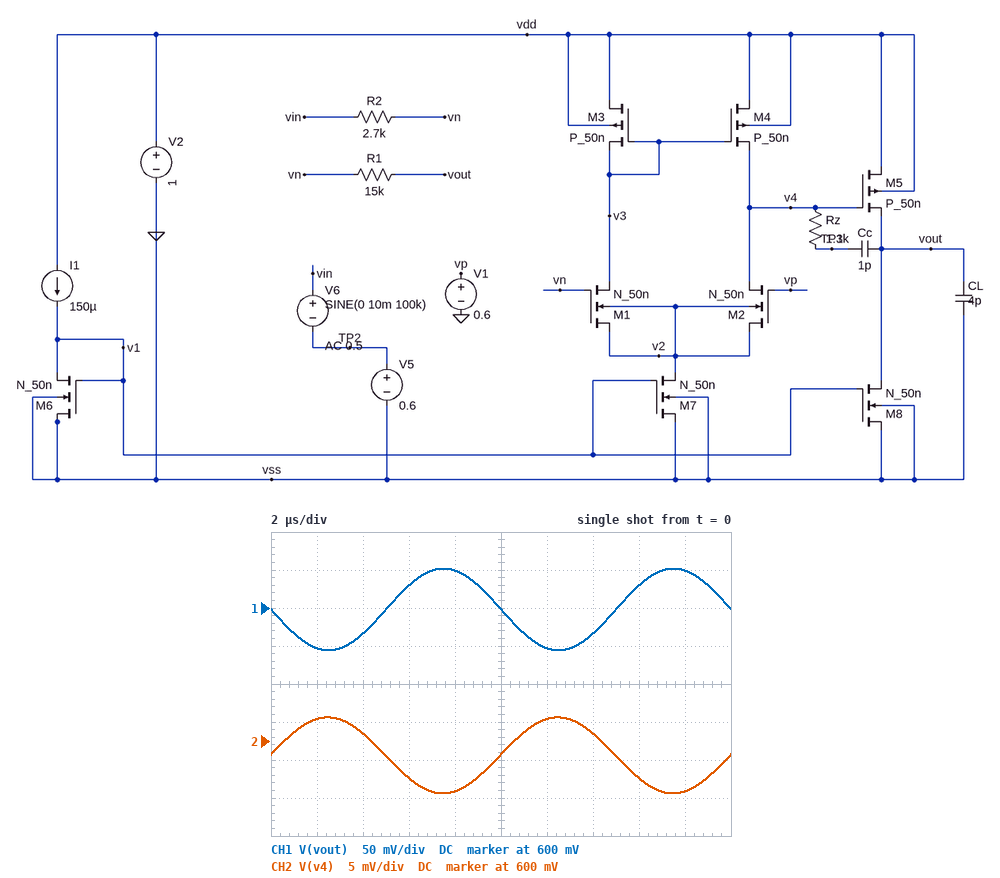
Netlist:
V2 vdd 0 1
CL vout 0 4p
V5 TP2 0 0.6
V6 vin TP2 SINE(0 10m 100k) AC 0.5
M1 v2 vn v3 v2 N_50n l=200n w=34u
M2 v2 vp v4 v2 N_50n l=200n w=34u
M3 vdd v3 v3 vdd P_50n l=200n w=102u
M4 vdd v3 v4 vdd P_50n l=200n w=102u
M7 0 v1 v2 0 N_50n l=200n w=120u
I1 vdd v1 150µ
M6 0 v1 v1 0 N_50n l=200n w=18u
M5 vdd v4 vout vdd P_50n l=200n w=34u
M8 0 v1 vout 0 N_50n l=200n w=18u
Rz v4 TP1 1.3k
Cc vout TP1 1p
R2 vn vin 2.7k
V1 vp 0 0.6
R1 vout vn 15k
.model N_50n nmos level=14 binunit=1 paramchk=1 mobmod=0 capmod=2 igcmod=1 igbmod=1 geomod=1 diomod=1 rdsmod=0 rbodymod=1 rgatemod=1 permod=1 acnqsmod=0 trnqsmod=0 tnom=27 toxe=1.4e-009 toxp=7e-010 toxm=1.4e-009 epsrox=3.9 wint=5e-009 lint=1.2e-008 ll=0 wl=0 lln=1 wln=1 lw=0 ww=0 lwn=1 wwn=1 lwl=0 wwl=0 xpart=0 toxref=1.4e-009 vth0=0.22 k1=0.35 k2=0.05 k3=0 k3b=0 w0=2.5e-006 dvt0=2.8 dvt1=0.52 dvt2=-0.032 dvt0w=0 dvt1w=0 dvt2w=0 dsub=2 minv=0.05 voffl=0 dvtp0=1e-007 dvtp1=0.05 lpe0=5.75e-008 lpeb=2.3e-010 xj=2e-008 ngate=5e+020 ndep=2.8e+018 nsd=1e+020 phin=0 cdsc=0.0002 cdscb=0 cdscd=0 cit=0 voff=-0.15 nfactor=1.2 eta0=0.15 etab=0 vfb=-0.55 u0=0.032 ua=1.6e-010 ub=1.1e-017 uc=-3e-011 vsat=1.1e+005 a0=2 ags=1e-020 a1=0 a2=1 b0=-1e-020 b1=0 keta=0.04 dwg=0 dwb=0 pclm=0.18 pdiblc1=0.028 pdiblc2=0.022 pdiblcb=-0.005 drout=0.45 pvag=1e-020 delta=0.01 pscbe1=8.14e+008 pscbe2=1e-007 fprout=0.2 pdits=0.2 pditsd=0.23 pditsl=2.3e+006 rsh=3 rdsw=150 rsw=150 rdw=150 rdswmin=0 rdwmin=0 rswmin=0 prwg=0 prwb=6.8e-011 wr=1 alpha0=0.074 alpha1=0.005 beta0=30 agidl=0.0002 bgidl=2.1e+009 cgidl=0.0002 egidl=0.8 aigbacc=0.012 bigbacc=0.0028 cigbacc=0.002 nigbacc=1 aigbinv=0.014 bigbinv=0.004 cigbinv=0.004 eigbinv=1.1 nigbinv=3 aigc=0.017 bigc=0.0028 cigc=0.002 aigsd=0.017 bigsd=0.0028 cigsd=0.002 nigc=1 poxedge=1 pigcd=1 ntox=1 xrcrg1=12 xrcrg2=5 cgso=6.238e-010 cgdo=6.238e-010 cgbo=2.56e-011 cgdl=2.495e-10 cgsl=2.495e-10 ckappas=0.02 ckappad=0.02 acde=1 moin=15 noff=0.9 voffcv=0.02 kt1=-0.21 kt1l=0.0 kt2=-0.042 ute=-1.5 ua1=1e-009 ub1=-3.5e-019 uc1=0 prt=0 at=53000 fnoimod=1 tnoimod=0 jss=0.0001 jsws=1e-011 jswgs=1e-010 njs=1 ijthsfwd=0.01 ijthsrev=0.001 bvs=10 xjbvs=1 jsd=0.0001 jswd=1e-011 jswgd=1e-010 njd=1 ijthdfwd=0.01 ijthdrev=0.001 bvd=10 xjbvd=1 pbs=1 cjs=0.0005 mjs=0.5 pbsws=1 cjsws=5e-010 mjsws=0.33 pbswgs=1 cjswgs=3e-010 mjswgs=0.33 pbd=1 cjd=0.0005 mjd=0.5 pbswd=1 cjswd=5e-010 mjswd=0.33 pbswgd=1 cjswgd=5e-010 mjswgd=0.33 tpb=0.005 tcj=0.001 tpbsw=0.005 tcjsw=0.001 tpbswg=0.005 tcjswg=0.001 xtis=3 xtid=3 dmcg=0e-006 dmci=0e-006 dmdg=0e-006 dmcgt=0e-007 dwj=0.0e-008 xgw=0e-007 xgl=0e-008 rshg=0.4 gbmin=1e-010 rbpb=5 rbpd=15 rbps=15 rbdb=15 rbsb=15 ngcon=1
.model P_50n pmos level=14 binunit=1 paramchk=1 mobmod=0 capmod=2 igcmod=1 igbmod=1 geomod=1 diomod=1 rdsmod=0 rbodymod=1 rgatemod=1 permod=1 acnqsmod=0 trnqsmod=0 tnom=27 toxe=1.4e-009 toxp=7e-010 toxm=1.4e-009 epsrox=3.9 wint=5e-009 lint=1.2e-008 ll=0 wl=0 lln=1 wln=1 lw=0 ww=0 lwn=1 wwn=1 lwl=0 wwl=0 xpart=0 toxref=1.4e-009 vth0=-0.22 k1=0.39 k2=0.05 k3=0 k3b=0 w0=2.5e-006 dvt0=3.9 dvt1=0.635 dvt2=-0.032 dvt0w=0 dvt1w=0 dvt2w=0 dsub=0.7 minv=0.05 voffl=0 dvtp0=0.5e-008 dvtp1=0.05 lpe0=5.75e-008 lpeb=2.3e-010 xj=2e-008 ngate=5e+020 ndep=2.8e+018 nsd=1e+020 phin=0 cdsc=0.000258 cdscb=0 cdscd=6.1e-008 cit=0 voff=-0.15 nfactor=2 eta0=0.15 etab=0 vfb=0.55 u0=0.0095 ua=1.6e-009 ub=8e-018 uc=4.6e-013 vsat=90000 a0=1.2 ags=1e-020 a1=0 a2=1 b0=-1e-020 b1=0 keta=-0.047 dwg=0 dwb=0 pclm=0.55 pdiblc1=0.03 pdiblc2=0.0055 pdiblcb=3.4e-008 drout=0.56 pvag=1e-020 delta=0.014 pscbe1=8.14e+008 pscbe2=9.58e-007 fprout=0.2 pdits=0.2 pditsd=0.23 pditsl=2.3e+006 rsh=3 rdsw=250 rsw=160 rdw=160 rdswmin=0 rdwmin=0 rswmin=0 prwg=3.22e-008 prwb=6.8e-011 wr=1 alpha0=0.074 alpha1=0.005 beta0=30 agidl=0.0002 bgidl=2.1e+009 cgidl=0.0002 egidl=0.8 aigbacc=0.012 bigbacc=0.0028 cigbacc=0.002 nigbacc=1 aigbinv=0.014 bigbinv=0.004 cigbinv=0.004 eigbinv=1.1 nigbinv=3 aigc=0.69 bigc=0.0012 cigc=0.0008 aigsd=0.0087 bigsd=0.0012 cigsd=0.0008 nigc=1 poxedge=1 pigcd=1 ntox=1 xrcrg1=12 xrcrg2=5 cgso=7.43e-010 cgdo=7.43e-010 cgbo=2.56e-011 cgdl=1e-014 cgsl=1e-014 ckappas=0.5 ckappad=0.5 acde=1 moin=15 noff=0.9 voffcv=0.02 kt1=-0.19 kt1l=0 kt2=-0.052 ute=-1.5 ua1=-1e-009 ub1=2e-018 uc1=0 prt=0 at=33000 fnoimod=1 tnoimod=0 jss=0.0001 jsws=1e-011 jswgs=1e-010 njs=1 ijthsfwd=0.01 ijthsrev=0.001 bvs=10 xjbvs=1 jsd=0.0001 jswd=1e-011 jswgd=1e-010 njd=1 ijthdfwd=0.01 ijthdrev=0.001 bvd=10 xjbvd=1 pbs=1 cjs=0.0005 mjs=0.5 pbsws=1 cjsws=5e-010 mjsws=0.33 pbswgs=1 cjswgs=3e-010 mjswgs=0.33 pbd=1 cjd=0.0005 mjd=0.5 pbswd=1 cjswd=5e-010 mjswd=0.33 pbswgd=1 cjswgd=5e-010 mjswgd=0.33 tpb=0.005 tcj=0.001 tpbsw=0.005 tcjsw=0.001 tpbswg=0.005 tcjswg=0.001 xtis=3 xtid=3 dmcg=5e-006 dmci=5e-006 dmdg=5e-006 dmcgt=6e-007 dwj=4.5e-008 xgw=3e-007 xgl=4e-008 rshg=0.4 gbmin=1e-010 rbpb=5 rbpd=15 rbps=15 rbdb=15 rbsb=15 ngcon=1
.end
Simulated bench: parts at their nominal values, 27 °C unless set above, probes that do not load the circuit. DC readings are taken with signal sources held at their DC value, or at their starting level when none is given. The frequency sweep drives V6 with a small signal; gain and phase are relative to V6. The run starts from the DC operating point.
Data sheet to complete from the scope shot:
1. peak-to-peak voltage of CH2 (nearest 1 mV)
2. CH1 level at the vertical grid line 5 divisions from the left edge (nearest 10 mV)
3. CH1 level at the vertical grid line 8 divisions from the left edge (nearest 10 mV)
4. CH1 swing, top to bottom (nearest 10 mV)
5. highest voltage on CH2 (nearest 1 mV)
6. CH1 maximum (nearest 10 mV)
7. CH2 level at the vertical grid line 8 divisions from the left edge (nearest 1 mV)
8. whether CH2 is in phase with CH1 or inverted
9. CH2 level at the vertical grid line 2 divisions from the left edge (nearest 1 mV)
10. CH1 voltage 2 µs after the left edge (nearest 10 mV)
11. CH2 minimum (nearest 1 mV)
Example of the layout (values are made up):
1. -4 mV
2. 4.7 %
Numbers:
1. 10 mV
2. 600 mV
3. 630 mV
4. 110 mV
5. 603 mV
6. 650 mV
7. 595 mV
8. inverted
9. 601 mV
10. 550 mV
11. 593 mV
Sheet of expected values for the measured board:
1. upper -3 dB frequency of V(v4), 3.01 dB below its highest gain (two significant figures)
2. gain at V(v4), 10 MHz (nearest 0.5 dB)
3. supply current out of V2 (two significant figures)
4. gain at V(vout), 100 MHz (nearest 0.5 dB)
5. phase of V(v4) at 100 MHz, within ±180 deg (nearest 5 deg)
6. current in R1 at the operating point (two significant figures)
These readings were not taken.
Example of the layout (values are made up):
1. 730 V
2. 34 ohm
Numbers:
1. 95 MHz
2. 1.5 dB
3. 1.2 mA
4. 7.5 dB
5. -60 deg
6. 100 nA
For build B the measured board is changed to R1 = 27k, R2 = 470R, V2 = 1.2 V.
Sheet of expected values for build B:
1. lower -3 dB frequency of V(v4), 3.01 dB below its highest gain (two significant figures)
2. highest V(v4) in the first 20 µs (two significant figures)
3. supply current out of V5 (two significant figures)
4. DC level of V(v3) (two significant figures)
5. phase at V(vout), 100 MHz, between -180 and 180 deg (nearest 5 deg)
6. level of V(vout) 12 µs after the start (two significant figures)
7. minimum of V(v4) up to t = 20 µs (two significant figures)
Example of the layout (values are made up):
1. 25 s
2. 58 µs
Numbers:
1. 5.8 MHz
2. 840 mV
3. 170 nA
4. 800 mV
5. 25 deg
6. 160 mV
7. 760 mV
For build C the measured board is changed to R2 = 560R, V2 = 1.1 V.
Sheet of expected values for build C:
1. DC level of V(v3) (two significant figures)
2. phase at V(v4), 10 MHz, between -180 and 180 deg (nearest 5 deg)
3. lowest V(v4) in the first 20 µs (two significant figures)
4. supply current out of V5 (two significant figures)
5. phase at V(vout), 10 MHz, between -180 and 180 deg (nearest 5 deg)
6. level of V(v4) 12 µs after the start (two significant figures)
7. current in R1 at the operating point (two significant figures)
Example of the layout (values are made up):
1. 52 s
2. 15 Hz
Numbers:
1. 700 mV
2. 30 deg
3. 680 mV
4. 310 nA
5. 145 deg
6. 720 mV
7. 300 nA
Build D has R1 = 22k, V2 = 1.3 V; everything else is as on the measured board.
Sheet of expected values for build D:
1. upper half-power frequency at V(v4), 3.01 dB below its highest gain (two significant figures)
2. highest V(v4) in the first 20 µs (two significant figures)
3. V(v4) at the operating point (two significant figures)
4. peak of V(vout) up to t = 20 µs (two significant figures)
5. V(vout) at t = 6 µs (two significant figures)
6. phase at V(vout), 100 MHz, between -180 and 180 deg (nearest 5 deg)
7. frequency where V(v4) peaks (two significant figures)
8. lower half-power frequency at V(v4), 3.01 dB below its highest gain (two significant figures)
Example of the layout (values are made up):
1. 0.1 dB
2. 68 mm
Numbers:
1. 90 MHz
2. 910 mV
3. 900 mV
4. 680 mV
5. 650 mV
6. 20 deg
7. 53 MHz
8. 32 MHz
